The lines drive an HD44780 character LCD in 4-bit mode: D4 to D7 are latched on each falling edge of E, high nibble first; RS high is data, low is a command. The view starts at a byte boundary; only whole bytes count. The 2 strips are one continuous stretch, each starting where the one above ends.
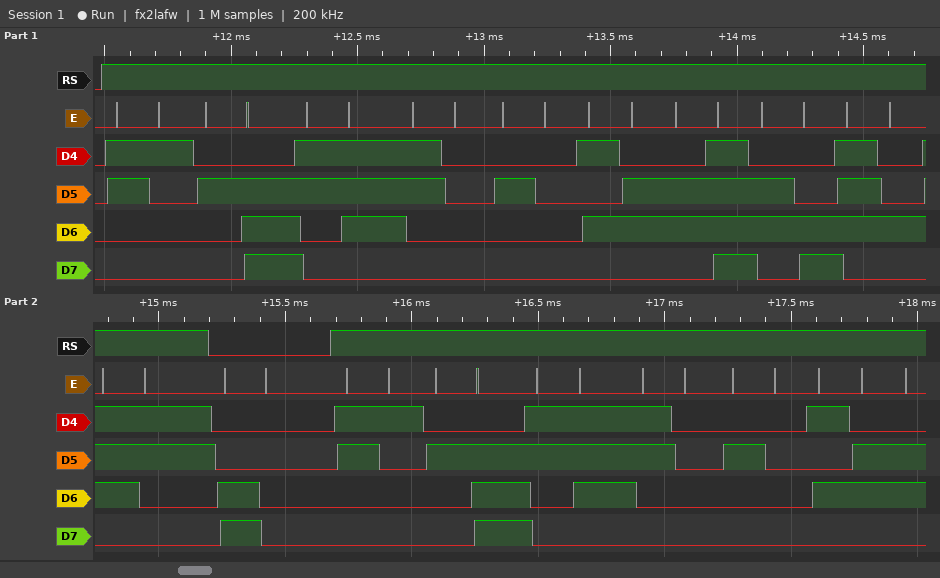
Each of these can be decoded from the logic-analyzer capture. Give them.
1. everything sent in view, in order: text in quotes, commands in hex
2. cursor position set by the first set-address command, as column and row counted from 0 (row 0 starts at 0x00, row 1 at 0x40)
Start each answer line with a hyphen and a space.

- "1.70 Volts" 0xC0 "1.70 V"
- column 0, row 1
